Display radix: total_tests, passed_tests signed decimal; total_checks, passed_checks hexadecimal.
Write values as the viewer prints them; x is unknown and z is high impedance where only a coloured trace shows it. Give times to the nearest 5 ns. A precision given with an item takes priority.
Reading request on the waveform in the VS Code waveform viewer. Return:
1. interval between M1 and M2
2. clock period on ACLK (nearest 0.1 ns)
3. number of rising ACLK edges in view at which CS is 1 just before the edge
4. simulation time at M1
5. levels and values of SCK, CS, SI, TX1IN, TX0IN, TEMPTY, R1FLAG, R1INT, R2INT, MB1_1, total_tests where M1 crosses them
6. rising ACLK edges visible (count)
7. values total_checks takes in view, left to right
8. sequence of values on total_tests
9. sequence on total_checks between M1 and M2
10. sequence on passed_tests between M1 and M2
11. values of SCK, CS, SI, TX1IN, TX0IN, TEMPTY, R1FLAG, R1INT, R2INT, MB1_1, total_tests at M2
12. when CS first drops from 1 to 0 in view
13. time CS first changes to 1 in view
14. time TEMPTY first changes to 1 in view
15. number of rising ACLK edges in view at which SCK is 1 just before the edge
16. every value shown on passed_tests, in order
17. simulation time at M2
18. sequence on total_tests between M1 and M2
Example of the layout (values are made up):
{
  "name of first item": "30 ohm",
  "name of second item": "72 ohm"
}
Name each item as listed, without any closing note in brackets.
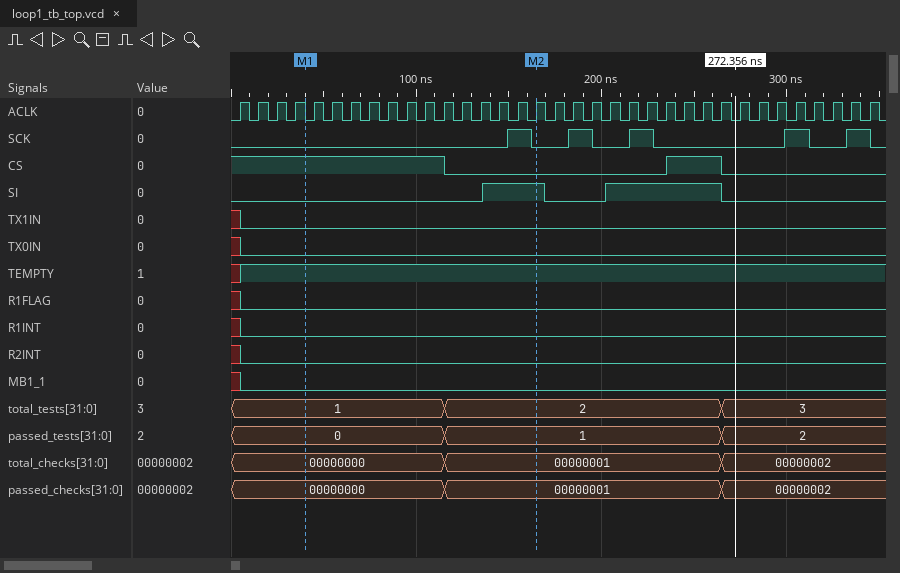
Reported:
{
  "interval between M1 and M2": "125 ns",
  "clock period on ACLK": "10 ns",
  "number of rising ACLK edges in view at which CS is 1 just before the edge": "15",
  "simulation time at M1": "40 ns",
  "levels and values of SCK, CS, SI, TX1IN, TX0IN, TEMPTY, R1FLAG, R1INT, R2INT, MB1_1, total_tests where M1 crosses them": "SCK=0, CS=1, SI=0, TX1IN=0, TX0IN=0, TEMPTY=1, R1FLAG=0, R1INT=0, R2INT=0, MB1_1=0, total_tests=1",
  "rising ACLK edges visible": "35",
  "values total_checks takes in view, left to right": "00000000, 00000001, 00000002",
  "sequence of values on total_tests": "1, 2, 3",
  "sequence on total_checks between M1 and M2": "00000000, 00000001",
  "sequence on passed_tests between M1 and M2": "0, 1",
  "values of SCK, CS, SI, TX1IN, TX0IN, TEMPTY, R1FLAG, R1INT, R2INT, MB1_1, total_tests at M2": "SCK=0, CS=0, SI=1, TX1IN=0, TX0IN=0, TEMPTY=1, R1FLAG=0, R1INT=0, R2INT=0, MB1_1=0, total_tests=2",
  "when CS first drops from 1 to 0 in view": "115 ns",
  "time CS first changes to 1 in view": "235 ns",
  "time TEMPTY first changes to 1 in view": "5 ns",
  "number of rising ACLK edges in view at which SCK is 1 just before the edge": "7",
  "every value shown on passed_tests, in order": "0, 1, 2",
  "simulation time at M2": "165 ns",
  "sequence on total_tests between M1 and M2": "1, 2"
}
